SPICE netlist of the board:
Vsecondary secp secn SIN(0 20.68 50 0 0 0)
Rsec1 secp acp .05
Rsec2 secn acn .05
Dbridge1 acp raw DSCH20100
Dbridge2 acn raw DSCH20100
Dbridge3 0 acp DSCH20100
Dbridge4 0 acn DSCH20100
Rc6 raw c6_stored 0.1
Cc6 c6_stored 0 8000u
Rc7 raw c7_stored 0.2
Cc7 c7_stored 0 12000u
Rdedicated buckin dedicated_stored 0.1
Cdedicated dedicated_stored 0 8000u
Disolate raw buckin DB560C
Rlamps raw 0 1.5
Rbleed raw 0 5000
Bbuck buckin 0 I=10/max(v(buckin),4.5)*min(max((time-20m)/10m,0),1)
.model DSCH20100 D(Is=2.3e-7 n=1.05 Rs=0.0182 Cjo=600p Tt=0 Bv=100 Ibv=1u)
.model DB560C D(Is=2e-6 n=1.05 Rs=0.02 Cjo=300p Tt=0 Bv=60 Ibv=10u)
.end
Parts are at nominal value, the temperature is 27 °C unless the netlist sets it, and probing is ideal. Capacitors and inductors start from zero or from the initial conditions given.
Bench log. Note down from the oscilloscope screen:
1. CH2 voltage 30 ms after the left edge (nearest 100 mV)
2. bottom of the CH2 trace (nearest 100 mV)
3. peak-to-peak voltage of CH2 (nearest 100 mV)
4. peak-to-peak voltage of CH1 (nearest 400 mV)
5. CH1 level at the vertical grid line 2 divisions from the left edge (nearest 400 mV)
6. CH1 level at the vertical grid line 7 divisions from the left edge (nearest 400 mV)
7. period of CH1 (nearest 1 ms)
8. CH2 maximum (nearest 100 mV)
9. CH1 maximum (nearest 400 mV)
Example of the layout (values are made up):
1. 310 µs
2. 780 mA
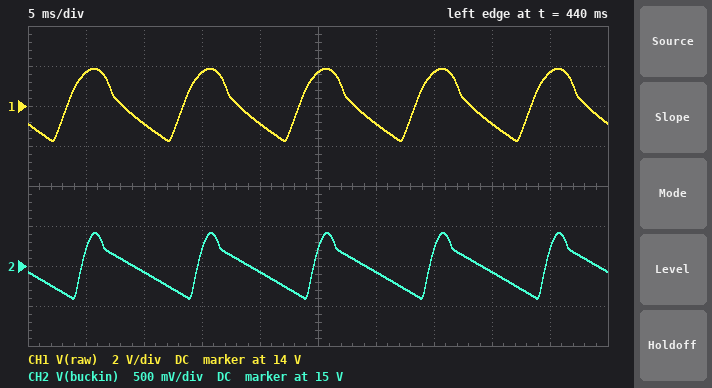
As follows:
1. 14.9 V
2. 14.6 V
3. 800 mV
4. 3.6 V
5. 13.2 V
6. 15.6 V
7. 10 ms
8. 15.4 V
9. 16.0 V
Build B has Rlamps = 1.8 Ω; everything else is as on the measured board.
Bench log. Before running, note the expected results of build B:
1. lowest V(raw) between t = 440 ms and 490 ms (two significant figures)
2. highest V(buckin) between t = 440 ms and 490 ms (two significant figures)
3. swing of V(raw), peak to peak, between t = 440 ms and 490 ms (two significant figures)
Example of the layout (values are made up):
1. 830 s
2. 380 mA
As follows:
1. 13 V
2. 16 V
3. 3.3 V
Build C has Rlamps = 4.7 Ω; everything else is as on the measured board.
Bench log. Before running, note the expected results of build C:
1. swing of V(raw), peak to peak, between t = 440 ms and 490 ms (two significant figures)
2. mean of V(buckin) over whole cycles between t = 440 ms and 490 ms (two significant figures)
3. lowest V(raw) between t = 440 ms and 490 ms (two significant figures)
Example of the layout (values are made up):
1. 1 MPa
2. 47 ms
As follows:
1. 1.8 V
2. 17 V
3. 16 V
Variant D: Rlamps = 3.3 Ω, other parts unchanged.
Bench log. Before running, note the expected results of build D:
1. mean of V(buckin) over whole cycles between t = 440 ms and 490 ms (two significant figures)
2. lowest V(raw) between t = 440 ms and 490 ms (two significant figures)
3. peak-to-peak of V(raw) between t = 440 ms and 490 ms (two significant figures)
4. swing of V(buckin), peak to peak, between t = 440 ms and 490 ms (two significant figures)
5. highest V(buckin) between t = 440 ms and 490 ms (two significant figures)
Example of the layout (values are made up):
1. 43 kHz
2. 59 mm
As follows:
1. 16 V
2. 15 V
3. 2.3 V
4. 760 mV
5. 17 V
